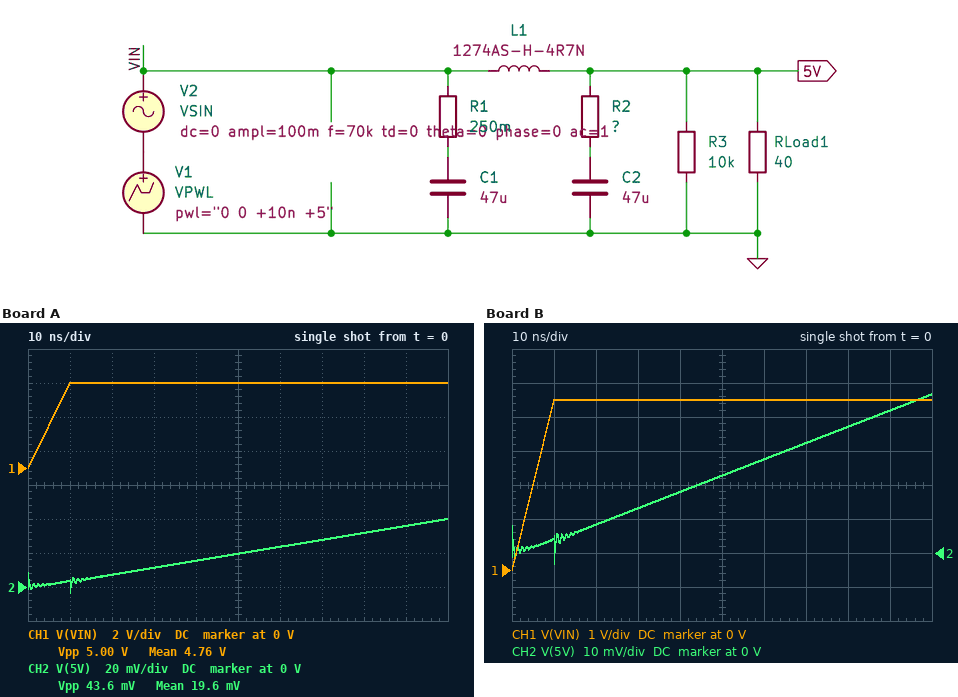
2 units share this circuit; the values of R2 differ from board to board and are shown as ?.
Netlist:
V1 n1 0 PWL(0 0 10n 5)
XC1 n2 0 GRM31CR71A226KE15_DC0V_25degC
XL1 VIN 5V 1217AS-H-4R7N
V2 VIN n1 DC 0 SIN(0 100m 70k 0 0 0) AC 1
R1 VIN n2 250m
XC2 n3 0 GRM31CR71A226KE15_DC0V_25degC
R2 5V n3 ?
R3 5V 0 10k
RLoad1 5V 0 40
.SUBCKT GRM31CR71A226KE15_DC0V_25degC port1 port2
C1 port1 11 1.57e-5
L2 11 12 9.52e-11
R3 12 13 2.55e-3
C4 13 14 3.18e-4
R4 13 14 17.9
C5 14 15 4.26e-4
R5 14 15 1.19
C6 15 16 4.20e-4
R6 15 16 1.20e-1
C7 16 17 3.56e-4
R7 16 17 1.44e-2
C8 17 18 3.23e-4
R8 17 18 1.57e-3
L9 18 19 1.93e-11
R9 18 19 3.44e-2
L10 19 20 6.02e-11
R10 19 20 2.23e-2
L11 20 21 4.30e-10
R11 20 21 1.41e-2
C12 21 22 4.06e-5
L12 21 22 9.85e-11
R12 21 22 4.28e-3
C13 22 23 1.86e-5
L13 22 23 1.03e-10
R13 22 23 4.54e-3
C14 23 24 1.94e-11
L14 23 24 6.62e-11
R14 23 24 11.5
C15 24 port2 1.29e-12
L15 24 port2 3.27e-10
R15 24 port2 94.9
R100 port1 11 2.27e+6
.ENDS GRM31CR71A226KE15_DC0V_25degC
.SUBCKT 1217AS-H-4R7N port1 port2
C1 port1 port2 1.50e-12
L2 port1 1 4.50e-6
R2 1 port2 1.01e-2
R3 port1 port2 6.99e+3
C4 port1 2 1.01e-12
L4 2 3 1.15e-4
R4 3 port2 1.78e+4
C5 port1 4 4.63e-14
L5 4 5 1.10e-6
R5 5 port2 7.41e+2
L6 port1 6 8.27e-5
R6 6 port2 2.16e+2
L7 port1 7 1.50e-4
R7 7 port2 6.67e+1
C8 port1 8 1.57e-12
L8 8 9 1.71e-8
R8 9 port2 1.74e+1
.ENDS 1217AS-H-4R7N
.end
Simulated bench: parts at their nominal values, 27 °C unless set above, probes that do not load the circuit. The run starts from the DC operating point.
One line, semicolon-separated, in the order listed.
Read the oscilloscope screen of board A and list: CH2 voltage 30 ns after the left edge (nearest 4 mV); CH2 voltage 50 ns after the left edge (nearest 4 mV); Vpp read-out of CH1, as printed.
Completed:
12 mV; 20 mV; 5.00 V
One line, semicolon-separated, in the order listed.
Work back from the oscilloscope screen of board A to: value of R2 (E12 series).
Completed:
0.33 Ω
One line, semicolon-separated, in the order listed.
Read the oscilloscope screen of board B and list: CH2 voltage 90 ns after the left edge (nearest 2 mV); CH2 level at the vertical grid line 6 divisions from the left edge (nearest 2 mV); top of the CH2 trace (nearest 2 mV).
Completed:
42 mV; 28 mV; 46 mV
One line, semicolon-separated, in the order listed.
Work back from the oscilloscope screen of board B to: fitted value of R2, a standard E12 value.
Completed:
0.39 Ω
